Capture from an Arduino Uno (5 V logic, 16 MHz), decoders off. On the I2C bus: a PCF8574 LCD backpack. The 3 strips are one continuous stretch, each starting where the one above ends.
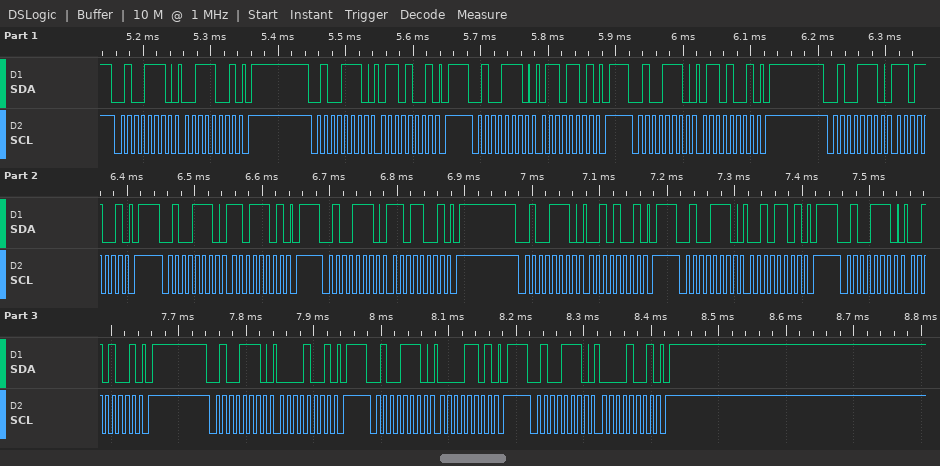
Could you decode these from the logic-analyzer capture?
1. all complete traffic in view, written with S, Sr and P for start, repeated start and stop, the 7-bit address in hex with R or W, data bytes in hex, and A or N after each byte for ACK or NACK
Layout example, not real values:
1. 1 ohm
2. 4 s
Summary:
1. S 27W A 39 A P S 27W A 69 A P S 27W A 6D A P S 27W A 69 A P S 27W A D9 A P S 27W A DD A P S 27W A D9 A P S 27W A 29 A P S 27W A 2D A P S 27W A 29 A P S 27W A 09 A P S 27W A 0D A P S 27W A 09 A P
